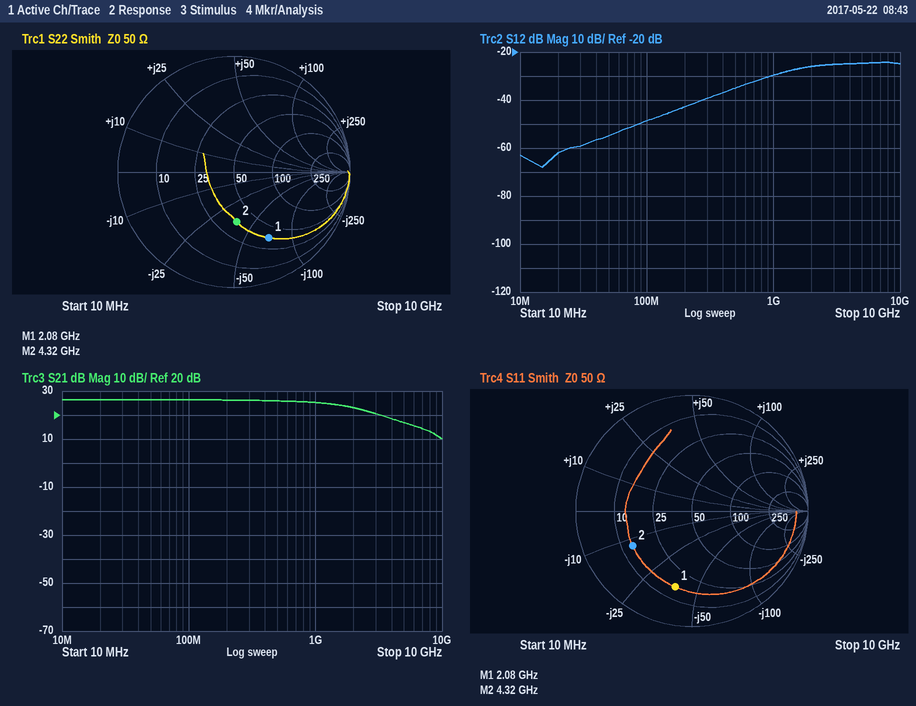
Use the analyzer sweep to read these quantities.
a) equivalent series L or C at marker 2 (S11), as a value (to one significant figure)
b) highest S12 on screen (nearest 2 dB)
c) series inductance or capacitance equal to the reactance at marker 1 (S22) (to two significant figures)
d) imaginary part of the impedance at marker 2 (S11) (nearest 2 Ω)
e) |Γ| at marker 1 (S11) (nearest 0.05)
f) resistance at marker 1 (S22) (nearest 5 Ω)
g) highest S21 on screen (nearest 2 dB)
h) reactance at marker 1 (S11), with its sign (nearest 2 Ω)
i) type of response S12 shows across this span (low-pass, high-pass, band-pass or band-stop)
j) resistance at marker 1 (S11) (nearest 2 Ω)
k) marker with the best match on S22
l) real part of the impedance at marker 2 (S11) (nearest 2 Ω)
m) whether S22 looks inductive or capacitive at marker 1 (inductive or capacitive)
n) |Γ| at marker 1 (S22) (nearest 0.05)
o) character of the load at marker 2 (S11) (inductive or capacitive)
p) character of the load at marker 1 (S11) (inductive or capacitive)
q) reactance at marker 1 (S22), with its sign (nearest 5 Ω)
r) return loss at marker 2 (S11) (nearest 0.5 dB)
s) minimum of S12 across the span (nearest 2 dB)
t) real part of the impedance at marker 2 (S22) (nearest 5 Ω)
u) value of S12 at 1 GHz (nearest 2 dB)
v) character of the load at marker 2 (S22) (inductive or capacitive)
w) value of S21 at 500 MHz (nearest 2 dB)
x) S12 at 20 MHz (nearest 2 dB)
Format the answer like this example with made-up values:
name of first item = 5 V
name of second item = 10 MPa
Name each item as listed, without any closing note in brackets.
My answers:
equivalent series L or C at marker 2 (S11), as a value = 3 pF
highest S12 on screen = -24 dB
series inductance or capacitance equal to the reactance at marker 1 (S22) = 1.1 pF
imaginary part of the impedance at marker 2 (S11) = -12 Ω
|Γ| at marker 1 (S11) = 0.65
resistance at marker 1 (S22) = 35 Ω
highest S21 on screen = 26 dB
reactance at marker 1 (S11), with its sign = -38 Ω
type of response S12 shows across this span = high-pass
resistance at marker 1 (S11) = 16 Ω
marker with the best match on S22 = marker 2
real part of the impedance at marker 2 (S11) = 14 Ω
whether S22 looks inductive or capacitive at marker 1 = capacitive
|Γ| at marker 1 (S22) = 0.65
character of the load at marker 2 (S11) = capacitive
character of the load at marker 1 (S11) = capacitive
reactance at marker 1 (S22), with its sign = -70 Ω
return loss at marker 2 (S11) = 4.5 dB
minimum of S12 across the span = -68 dB
real part of the impedance at marker 2 (S22) = 35 Ω
value of S12 at 1 GHz = -30 dB
character of the load at marker 2 (S22) = capacitive
value of S21 at 500 MHz = 26 dB
S12 at 20 MHz = -62 dB
